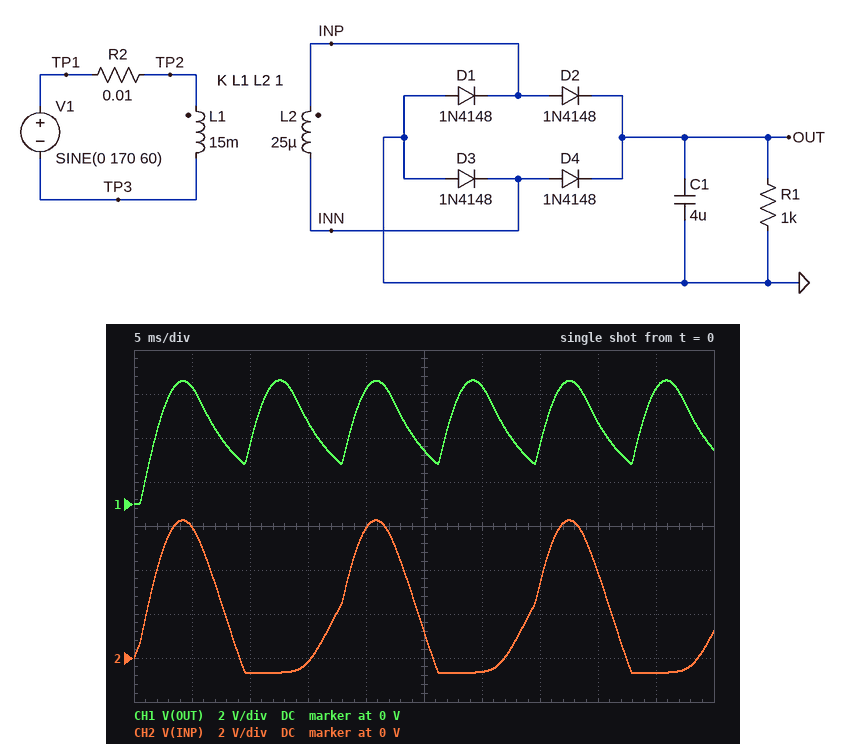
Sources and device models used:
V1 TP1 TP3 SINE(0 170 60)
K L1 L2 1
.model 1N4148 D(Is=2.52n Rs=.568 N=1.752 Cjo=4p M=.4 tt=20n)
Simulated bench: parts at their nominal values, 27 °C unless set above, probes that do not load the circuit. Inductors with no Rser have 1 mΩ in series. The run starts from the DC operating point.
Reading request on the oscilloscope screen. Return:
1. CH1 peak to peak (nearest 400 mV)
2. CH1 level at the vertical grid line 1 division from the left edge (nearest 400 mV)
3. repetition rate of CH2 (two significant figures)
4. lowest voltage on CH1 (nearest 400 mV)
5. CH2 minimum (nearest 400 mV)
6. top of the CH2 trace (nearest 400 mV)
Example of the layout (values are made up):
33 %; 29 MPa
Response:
5.6 V; 5.2 V; 60 Hz; 0 V; -800 mV; 6.4 V
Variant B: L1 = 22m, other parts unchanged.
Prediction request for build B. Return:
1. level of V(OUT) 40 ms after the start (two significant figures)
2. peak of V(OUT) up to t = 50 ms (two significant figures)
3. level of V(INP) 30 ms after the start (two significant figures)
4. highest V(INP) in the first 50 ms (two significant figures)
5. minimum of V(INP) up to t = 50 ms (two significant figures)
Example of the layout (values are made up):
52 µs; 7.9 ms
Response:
2.9 V; 4.4 V; -620 mV; 5.1 V; -690 mV
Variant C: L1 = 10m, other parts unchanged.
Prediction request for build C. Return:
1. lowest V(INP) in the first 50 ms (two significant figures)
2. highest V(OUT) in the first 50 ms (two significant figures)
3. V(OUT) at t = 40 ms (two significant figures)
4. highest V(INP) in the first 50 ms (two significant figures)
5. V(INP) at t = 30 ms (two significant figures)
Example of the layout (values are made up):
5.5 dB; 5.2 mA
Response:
-710 mV; 7.2 V; 4.7 V; 7.8 V; -640 mV
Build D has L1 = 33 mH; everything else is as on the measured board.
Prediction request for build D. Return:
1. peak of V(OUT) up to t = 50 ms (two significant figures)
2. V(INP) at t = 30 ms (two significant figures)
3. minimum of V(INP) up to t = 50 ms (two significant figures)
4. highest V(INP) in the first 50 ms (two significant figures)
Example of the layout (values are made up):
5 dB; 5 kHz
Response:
3.4 V; -610 mV; -680 mV; 4.0 V
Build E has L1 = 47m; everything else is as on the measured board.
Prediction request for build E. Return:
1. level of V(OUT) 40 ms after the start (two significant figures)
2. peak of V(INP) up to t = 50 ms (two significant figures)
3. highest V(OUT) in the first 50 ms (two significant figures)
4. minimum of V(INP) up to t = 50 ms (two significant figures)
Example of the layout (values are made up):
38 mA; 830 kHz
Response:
1.8 V; 3.3 V; 2.7 V; -670 mV
